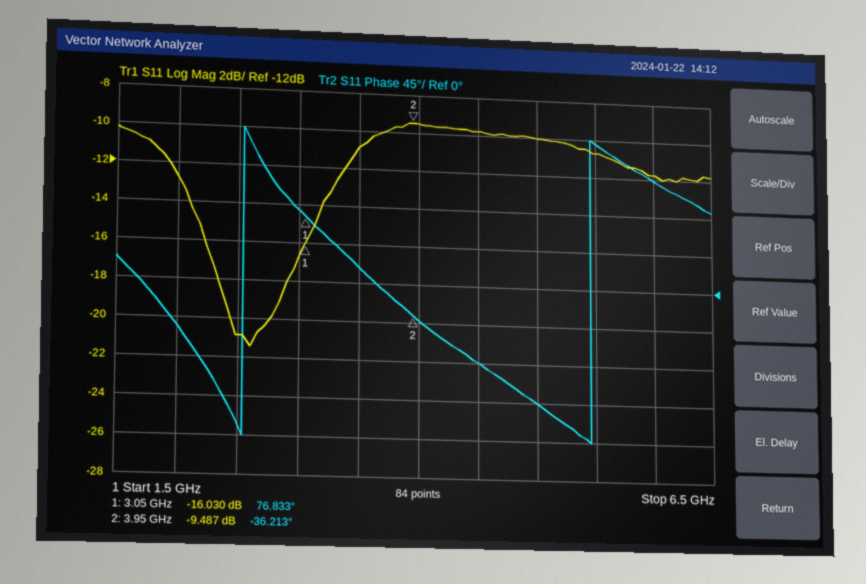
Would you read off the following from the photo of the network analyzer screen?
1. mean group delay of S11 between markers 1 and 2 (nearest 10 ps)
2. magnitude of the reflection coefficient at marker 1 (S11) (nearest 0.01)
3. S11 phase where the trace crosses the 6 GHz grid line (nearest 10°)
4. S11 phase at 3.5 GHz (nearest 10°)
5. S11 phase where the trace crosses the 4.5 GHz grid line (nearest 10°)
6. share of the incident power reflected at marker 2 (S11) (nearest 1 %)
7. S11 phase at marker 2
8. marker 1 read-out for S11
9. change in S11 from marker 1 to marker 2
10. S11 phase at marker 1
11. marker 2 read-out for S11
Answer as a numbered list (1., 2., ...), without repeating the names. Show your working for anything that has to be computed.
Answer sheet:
1. −(-36.213° − (76.833°))/(360° × 900 MHz) ≈ 349 ps, so 350 ps to the nearest 10 ps
2. 10^(-16.03/20) ≈ 0.16
3. 130°
4. 20°
5. -90°
6. 10^(-9.487/10) ≈ 11 %
7. -36.213°
8. -16.030 dB
9. -9.487 − (-16.03) = 6.543 dB
10. 76.833°
11. -9.487 dB
